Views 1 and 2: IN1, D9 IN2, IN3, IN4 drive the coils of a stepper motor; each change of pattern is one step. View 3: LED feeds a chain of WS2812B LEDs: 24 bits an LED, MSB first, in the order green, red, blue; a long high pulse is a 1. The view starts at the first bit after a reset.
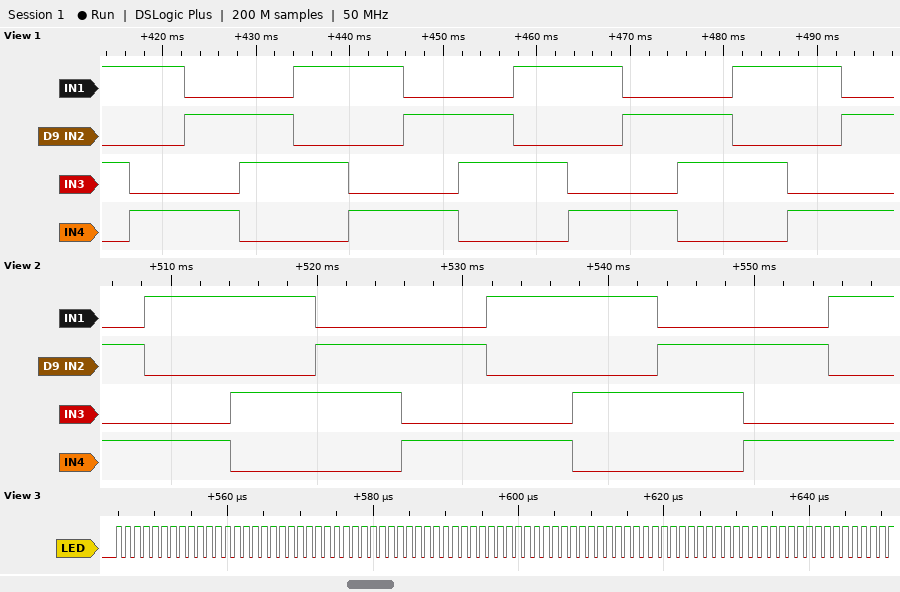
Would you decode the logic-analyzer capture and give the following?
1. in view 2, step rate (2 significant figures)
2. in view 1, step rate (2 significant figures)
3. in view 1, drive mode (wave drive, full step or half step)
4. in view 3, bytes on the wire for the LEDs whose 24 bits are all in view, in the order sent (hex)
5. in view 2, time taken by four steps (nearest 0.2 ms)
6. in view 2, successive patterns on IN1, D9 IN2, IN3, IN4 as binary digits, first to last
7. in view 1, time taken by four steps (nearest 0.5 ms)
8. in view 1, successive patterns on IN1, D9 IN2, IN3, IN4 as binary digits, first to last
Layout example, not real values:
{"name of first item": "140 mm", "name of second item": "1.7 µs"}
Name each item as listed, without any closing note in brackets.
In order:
{"in view 2, step rate": "170 steps/s", "in view 1, step rate": "170 steps/s", "in view 1, drive mode": "full step", "in view 3, bytes on the wire for the LEDs whose 24 bits are all in view, in the order sent": "FF FF FF FF FF FF FF FF FF", "in view 2, time taken by four steps": "23.4 ms", "in view 2, successive patterns on IN1, D9 IN2, IN3, IN4 as binary digits, first to last": "0101 1001 1010 0110 0101 1001 1010 0110 0101 1001", "in view 1, time taken by four steps": "23.5 ms", "in view 1, successive patterns on IN1, D9 IN2, IN3, IN4 as binary digits, first to last": "1010 1001 0101 0110 1010 1001 0101 0110 1010 1001 0101 0110 1010 1001 0101"}
